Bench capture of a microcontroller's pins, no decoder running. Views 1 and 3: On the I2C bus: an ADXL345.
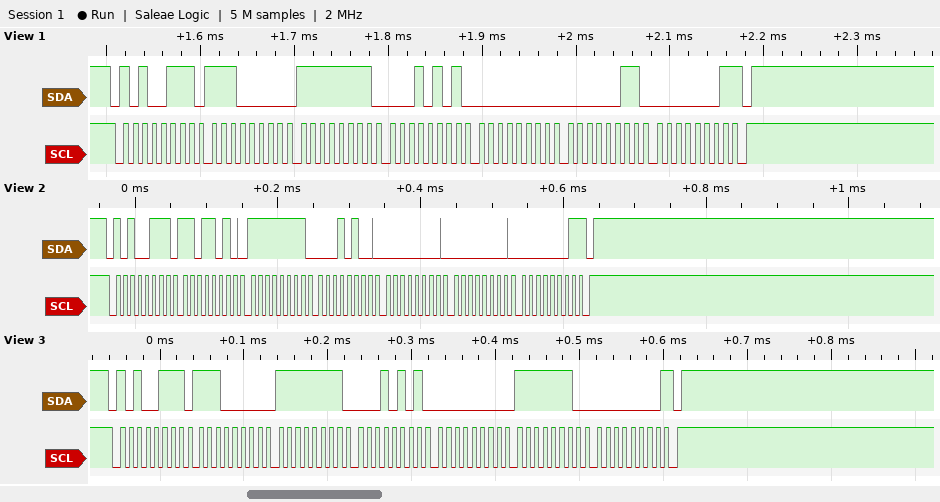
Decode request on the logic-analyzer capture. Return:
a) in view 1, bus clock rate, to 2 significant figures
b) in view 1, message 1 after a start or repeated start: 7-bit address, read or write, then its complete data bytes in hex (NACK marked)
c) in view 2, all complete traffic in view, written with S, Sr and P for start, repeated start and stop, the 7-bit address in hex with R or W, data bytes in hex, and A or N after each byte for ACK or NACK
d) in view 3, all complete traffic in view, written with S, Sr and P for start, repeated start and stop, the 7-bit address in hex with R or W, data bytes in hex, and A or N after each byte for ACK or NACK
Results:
100 kHz
0x53 read: E0 FF 15 00 03 01 NACK
S 53R A DA A FF A 14 A 00 A 00 A 01 N P
S 53R A E0 A FF A 15 A 00 A FE A 00 N P
